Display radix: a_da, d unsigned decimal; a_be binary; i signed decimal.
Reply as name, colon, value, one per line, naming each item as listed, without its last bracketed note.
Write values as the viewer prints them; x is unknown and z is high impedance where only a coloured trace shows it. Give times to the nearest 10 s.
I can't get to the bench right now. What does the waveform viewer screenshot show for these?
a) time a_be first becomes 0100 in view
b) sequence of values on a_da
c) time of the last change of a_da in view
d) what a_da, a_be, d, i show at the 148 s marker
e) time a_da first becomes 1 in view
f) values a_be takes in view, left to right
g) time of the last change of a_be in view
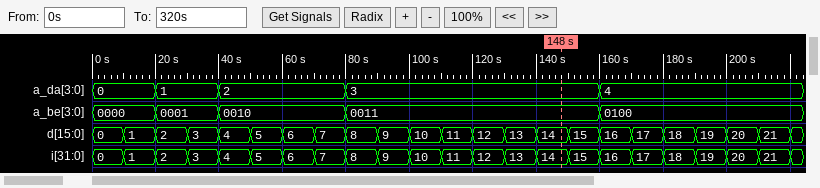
time a_be first becomes 0100 in view: 160 s
sequence of values on a_da: 0, 1, 2, 3, 4
time of the last change of a_da in view: 160 s
what a_da, a_be, d, i show at the 148 s marker: a_da=3, a_be=0011, d=14, i=14
time a_da first becomes 1 in view: 20 s
values a_be takes in view, left to right: 0000, 0001, 0010, 0011, 0100
time of the last change of a_be in view: 160 s
